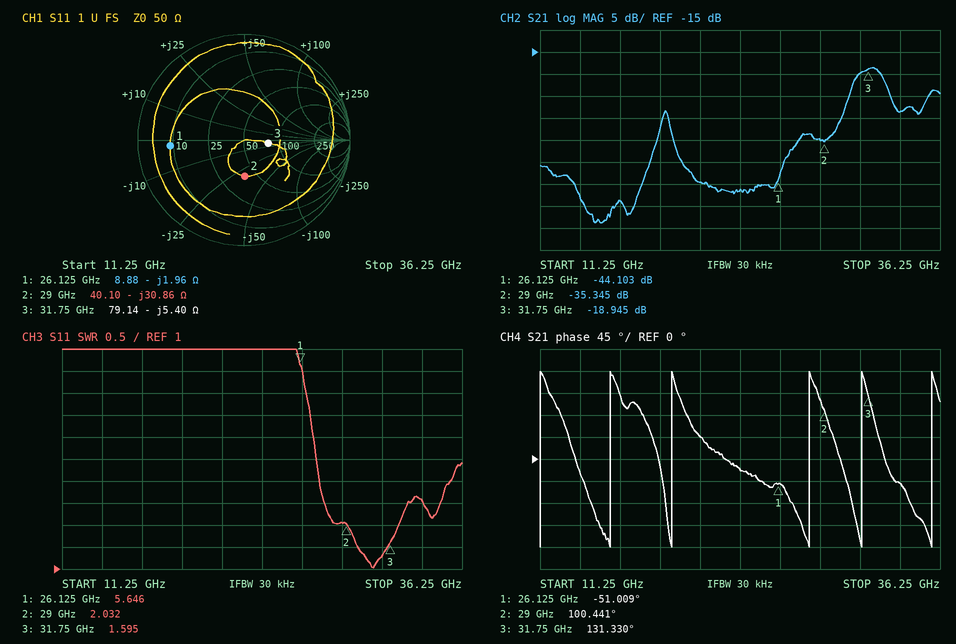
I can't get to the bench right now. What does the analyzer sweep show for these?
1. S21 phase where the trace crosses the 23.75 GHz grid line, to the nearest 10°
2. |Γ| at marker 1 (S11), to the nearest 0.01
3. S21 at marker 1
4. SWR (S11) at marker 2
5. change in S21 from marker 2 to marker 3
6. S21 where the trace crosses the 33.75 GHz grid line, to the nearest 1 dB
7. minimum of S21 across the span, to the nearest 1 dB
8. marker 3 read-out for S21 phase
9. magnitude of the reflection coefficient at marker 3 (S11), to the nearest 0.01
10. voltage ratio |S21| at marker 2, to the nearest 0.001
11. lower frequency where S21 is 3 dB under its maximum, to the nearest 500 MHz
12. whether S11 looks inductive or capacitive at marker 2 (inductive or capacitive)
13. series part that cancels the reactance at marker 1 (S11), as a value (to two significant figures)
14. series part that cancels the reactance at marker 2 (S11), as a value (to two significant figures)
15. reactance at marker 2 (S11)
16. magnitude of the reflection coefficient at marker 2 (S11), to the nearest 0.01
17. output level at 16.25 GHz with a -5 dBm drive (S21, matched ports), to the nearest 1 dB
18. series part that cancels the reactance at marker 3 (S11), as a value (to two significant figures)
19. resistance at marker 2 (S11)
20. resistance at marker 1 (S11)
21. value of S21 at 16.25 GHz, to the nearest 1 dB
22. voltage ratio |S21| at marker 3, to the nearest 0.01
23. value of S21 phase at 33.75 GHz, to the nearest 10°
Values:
-20°
0.70
-44.103 dB
2.032
16.400 dB
-29 dB
-54 dB
131.330°
0.23
0.017
31.0 GHz
capacitive
12 pH
170 pH
-30.86 Ω
0.34
-54 dBm
27 pH
40.10 Ω
8.88 Ω
-49 dB
0.11
-50°
